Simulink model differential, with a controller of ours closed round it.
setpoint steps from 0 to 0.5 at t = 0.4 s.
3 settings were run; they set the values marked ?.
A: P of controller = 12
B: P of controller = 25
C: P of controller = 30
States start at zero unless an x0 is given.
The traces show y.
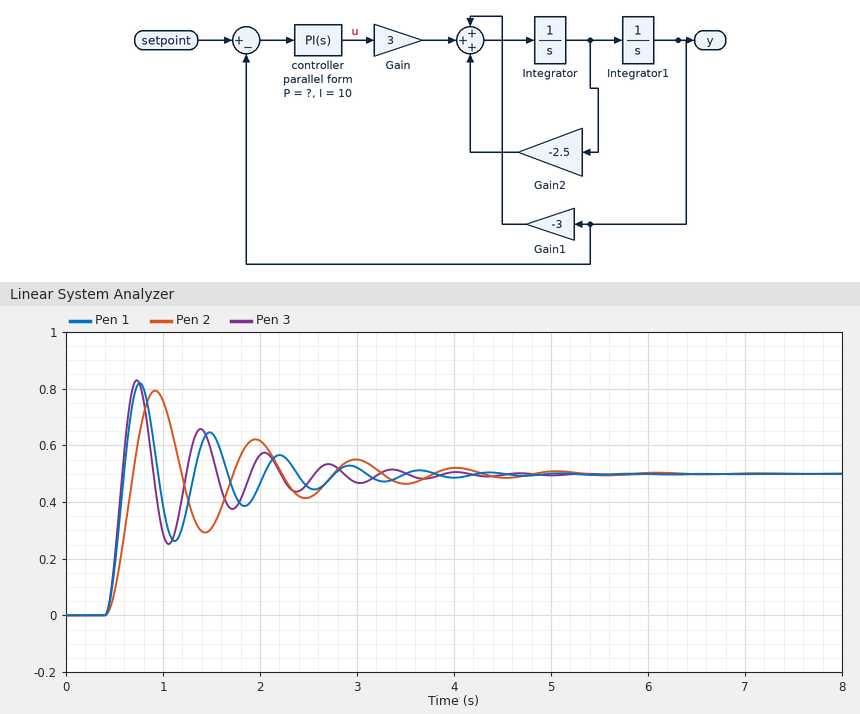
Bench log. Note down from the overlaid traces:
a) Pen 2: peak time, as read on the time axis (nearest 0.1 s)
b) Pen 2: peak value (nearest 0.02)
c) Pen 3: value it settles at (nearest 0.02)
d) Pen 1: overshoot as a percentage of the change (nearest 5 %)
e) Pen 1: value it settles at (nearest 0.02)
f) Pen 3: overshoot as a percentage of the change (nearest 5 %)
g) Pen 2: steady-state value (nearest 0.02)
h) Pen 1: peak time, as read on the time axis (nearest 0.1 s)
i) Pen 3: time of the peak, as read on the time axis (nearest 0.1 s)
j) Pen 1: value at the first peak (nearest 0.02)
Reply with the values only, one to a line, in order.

0.9 s
0.80
0.50
65 %
0.50
65 %
0.50
0.8 s
0.7 s
0.82
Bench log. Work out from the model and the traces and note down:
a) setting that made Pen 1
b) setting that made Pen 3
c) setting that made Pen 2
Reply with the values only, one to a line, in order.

B
C
A
